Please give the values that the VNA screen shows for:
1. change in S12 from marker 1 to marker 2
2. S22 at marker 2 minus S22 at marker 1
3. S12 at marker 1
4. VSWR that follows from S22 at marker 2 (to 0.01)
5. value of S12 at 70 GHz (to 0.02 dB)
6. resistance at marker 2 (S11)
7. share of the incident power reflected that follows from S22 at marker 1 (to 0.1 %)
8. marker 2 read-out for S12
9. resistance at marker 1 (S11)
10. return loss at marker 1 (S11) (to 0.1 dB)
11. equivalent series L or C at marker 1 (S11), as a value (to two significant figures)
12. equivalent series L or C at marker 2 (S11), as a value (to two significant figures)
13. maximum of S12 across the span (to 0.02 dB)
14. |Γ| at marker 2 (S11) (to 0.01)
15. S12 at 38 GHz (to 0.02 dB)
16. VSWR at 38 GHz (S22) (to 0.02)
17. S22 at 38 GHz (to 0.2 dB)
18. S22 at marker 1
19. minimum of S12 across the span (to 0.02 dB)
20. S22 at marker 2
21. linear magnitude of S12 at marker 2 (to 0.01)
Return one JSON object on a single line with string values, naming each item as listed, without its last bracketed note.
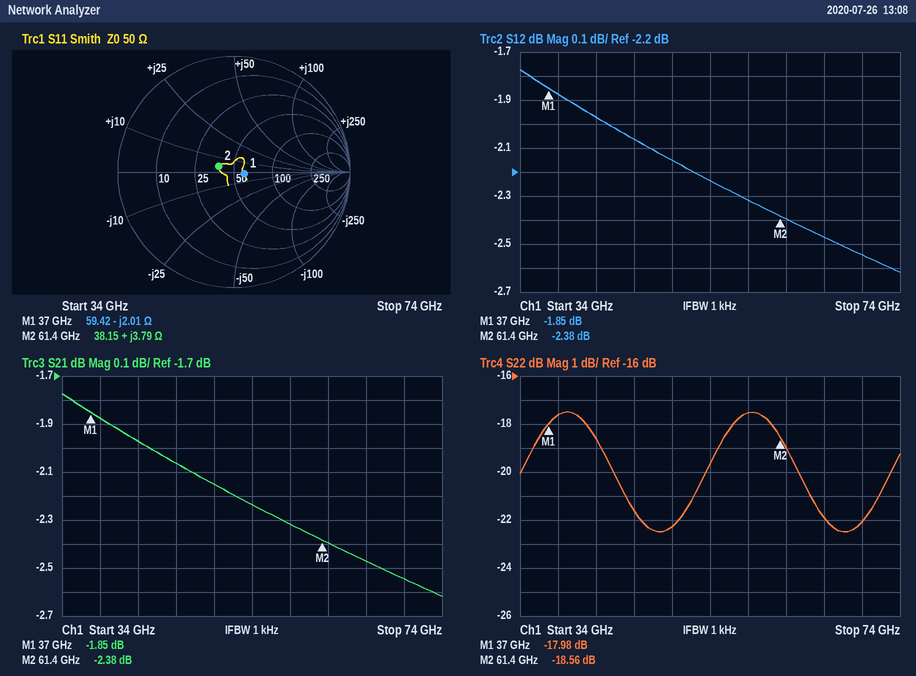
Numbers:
{"change in S12 from marker 1 to marker 2": "-0.53 dB", "S22 at marker 2 minus S22 at marker 1": "-0.58 dB", "S12 at marker 1": "-1.85 dB", "VSWR that follows from S22 at marker 2": "1.27", "value of S12 at 70 GHz": "-2.54 dB", "resistance at marker 2": "38.15 Ω", "share of the incident power reflected that follows from S22 at marker 1": "1.6 %", "marker 2 read-out for S12": "-2.38 dB", "resistance at marker 1": "59.42 Ω", "return loss at marker 1 (S11)": "21.1 dB", "equivalent series L or C at marker 1 (S11), as a value": "2.1 pF", "equivalent series L or C at marker 2 (S11), as a value": "9.8 pH", "maximum of S12 across the span": "-1.78 dB", "|Γ| at marker 2 (S11)": "0.14", "S12 at 38 GHz": "-1.88 dB", "VSWR at 38 GHz (S22)": "1.30", "S22 at 38 GHz": "-17.6 dB", "S22 at marker 1": "-17.98 dB", "minimum of S12 across the span": "-2.62 dB", "S22 at marker 2": "-18.56 dB", "linear magnitude of S12 at marker 2": "0.76"}
